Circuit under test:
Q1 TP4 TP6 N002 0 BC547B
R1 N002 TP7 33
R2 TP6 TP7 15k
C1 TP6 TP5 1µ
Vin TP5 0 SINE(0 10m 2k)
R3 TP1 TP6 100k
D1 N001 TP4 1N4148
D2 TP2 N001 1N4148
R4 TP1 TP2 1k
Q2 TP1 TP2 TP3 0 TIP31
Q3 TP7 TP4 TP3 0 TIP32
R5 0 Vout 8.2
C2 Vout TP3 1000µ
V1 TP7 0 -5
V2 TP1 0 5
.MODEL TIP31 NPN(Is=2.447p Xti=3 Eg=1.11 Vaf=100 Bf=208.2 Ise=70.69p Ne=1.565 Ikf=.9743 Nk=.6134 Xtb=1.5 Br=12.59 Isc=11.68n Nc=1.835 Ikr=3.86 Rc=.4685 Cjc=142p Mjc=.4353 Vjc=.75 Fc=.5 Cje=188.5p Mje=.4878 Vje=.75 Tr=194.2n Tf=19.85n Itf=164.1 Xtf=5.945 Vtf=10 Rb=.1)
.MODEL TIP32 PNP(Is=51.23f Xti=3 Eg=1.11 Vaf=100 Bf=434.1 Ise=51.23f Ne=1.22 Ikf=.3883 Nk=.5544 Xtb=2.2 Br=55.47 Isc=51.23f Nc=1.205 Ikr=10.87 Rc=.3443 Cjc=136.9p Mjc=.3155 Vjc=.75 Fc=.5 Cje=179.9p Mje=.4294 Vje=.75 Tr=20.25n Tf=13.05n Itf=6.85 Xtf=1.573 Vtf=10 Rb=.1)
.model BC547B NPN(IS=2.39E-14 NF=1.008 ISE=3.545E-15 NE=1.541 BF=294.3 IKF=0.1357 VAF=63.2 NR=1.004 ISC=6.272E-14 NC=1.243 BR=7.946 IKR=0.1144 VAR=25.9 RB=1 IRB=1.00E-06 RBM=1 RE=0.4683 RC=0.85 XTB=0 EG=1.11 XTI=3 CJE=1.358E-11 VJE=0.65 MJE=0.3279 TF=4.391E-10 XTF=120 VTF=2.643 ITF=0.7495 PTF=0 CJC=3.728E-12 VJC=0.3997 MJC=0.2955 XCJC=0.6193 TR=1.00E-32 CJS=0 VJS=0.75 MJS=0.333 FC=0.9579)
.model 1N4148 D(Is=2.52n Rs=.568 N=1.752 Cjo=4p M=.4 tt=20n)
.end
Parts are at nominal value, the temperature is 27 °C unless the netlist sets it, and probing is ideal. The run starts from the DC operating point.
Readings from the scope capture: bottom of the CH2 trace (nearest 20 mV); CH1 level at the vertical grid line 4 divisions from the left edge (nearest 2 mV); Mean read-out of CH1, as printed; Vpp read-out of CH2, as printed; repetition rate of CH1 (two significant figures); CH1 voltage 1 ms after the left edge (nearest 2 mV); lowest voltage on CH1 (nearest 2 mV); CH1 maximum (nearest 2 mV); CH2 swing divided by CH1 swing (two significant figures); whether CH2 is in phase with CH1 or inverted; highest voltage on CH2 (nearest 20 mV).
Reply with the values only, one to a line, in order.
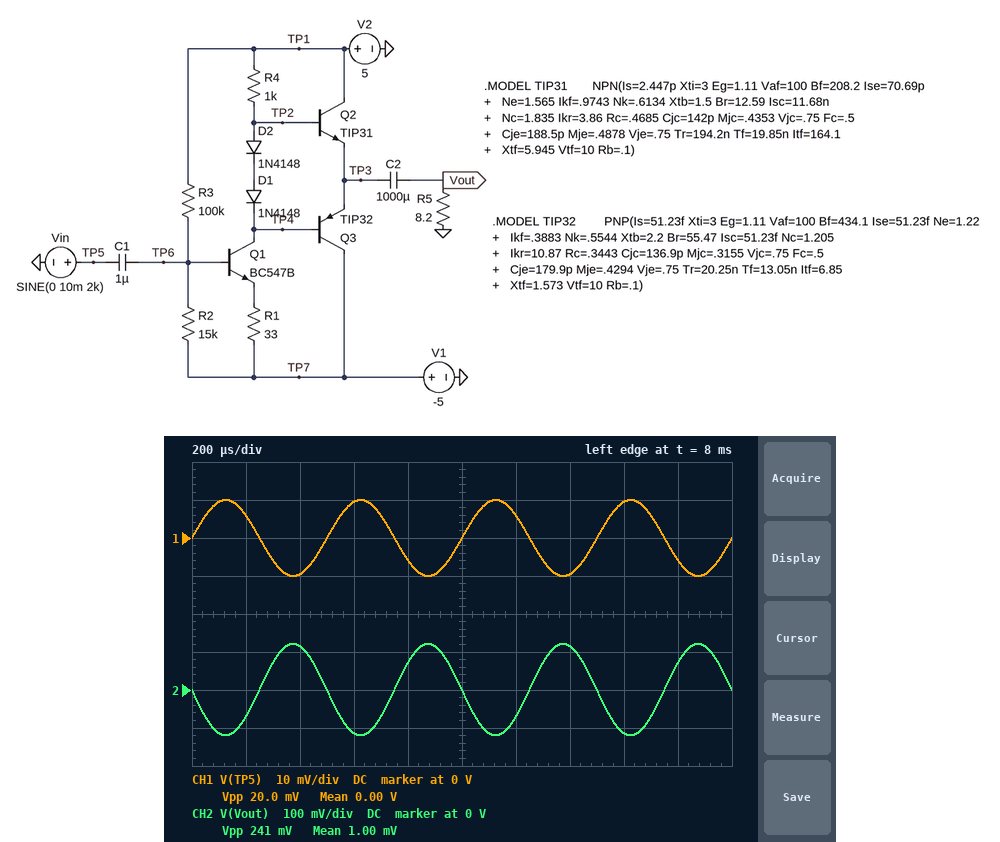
-120 mV
-6 mV
0.00 V
241 mV
2.0 kHz
0 V
-10 mV
10 mV
12
inverted
120 mV
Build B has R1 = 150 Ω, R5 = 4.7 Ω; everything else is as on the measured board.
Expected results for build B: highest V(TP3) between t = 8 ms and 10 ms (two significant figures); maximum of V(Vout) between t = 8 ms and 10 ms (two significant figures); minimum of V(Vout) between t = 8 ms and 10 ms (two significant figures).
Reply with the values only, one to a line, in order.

1.1 V
20 mV
-20 mV
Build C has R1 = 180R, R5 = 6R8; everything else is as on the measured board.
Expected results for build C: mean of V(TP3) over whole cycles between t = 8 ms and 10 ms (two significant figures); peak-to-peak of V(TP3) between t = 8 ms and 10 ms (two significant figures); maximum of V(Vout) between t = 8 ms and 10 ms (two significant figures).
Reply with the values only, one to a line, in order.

1.5 V
41 mV
21 mV
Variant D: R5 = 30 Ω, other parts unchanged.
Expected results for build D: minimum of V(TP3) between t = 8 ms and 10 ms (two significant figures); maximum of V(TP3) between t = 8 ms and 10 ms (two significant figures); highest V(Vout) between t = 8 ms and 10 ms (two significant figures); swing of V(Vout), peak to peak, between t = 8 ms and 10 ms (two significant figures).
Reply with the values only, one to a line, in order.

-3.3 V
-2.9 V
200 mV
390 mV
